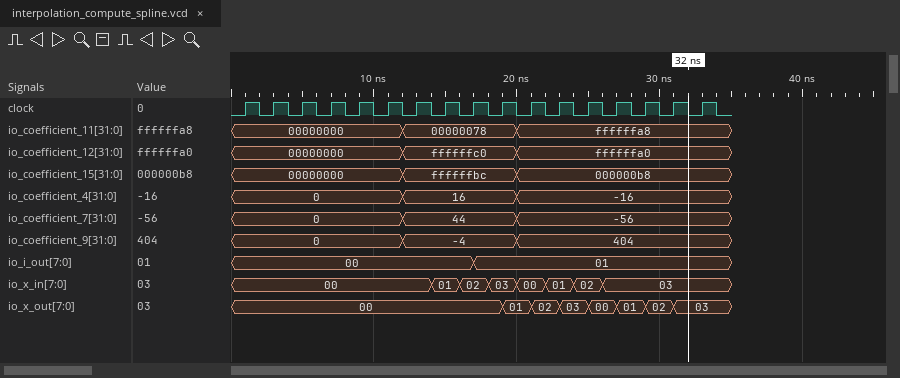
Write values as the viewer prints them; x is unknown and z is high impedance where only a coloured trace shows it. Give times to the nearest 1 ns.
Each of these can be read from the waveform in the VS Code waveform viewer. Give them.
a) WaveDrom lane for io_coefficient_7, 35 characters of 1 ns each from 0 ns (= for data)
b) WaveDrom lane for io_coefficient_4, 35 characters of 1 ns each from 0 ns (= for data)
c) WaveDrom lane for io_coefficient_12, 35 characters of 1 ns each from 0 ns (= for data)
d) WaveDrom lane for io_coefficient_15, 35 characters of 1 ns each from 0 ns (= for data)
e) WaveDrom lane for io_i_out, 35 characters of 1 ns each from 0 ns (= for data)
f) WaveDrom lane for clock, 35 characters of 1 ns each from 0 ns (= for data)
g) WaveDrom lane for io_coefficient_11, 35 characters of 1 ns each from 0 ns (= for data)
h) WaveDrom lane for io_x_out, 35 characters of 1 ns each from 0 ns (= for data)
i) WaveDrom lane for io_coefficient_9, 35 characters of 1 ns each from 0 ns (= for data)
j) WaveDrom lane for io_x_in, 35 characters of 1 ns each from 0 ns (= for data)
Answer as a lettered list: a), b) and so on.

a) {name: 'io_coefficient_7', wave: '=...........=.......=..............', data: '0 44 -56'}
b) {name: 'io_coefficient_4', wave: '=...........=.......=..............', data: '0 16 -16'}
c) {name: 'io_coefficient_12', wave: '=...........=.......=..............', data: '00000000 ffffffc0 ffffffa0'}
d) {name: 'io_coefficient_15', wave: '=...........=.......=..............', data: '00000000 ffffffbc 000000b8'}
e) {name: 'io_i_out', wave: '=................=.................', data: '00 01'}
f) {name: 'clock', wave: '01010101010101010101010101010101010'}
g) {name: 'io_coefficient_11', wave: '=...........=.......=..............', data: '00000000 00000078 ffffffa8'}
h) {name: 'io_x_out', wave: '=..................=.=.=.=.=.=.=...', data: '00 01 02 03 00 01 02 03'}
i) {name: 'io_coefficient_9', wave: '=...........=.......=..............', data: '0 -4 404'}
j) {name: 'io_x_in', wave: '=.............=.=.=.=.=.=.=........', data: '00 01 02 03 00 01 02 03'}
